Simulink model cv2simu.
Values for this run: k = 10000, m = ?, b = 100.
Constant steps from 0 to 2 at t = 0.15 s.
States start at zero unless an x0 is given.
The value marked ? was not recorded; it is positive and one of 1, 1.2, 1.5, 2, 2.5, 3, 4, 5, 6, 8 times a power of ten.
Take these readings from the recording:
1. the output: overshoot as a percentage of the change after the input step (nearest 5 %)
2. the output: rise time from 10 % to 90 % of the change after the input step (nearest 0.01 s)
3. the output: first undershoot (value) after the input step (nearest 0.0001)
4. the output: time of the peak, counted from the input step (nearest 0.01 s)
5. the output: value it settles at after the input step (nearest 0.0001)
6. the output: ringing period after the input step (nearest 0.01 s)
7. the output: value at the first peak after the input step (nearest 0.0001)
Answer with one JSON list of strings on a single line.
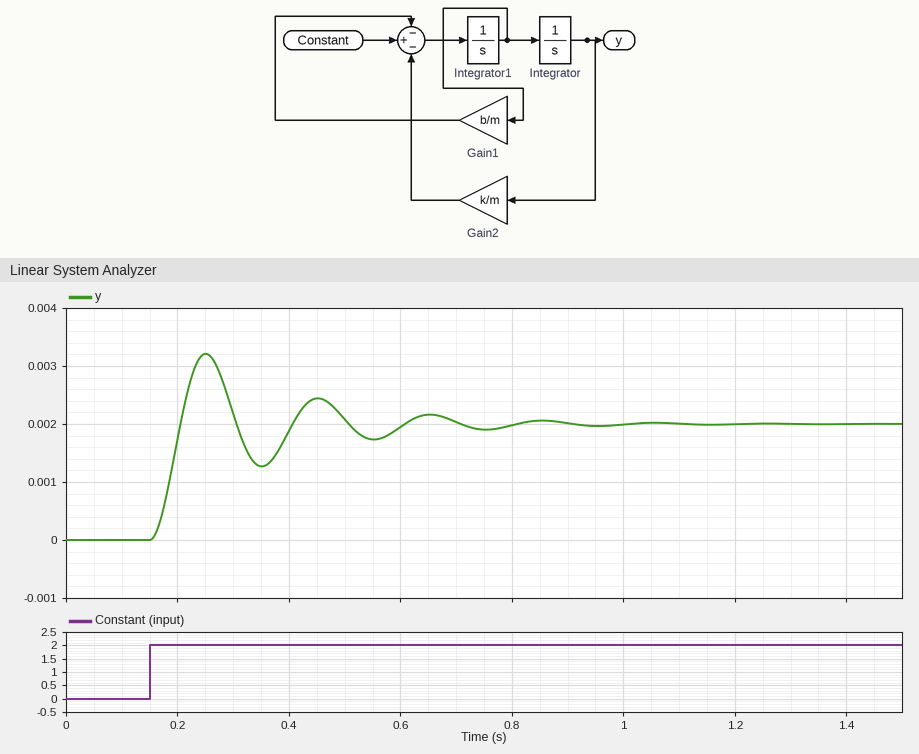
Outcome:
["60 %", "0.04 s", "0.0013", "0.10 s", "0.0020", "0.20 s", "0.0032"]
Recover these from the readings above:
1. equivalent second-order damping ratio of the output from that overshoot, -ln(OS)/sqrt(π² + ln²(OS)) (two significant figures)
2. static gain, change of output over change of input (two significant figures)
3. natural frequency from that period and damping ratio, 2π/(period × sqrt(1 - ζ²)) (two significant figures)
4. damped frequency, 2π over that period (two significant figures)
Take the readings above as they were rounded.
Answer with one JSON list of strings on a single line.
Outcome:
["0.16", "0.0010", "32 rad/s", "31 rad/s"]
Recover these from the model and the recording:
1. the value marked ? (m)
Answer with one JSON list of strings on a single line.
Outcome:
["10"]
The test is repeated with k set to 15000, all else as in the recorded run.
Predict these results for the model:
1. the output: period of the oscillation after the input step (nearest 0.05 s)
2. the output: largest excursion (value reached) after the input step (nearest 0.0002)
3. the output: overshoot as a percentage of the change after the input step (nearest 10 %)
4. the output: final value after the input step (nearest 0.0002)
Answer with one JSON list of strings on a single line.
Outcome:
["0.15 s", "0.0022", "70 %", "0.0014"]
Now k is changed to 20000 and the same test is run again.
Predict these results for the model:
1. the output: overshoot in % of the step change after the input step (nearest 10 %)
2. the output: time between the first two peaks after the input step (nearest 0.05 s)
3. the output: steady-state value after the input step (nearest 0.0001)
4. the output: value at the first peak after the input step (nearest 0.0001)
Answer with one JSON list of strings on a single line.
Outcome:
["70 %", "0.15 s", "0.0010", "0.0017"]
